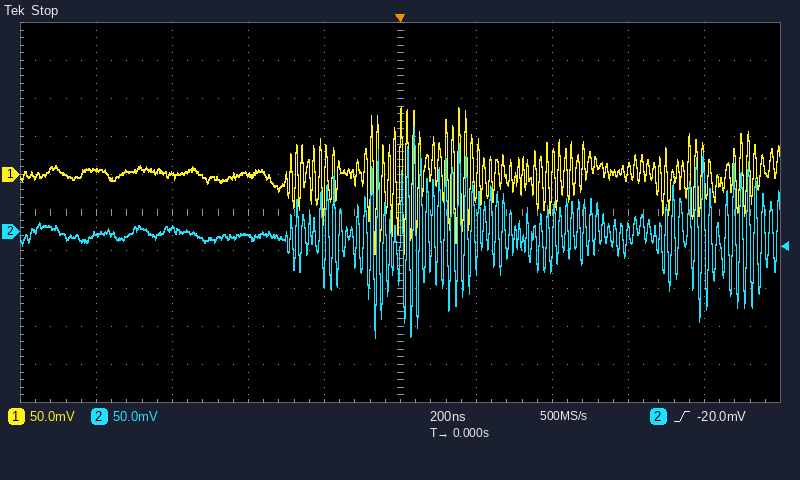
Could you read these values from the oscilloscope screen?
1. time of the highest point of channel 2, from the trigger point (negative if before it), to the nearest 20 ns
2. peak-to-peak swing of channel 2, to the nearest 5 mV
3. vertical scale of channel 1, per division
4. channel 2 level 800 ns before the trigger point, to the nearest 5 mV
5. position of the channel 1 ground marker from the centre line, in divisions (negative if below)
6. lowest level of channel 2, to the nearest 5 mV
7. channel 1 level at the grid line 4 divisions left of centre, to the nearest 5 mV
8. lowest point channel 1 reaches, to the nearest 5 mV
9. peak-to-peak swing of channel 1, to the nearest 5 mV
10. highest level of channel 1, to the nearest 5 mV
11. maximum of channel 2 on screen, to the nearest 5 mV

+40 ns
280 mV
50 mV
-5 mV
+1.0 div
-140 mV
5 mV
-105 mV
195 mV
90 mV
140 mV
